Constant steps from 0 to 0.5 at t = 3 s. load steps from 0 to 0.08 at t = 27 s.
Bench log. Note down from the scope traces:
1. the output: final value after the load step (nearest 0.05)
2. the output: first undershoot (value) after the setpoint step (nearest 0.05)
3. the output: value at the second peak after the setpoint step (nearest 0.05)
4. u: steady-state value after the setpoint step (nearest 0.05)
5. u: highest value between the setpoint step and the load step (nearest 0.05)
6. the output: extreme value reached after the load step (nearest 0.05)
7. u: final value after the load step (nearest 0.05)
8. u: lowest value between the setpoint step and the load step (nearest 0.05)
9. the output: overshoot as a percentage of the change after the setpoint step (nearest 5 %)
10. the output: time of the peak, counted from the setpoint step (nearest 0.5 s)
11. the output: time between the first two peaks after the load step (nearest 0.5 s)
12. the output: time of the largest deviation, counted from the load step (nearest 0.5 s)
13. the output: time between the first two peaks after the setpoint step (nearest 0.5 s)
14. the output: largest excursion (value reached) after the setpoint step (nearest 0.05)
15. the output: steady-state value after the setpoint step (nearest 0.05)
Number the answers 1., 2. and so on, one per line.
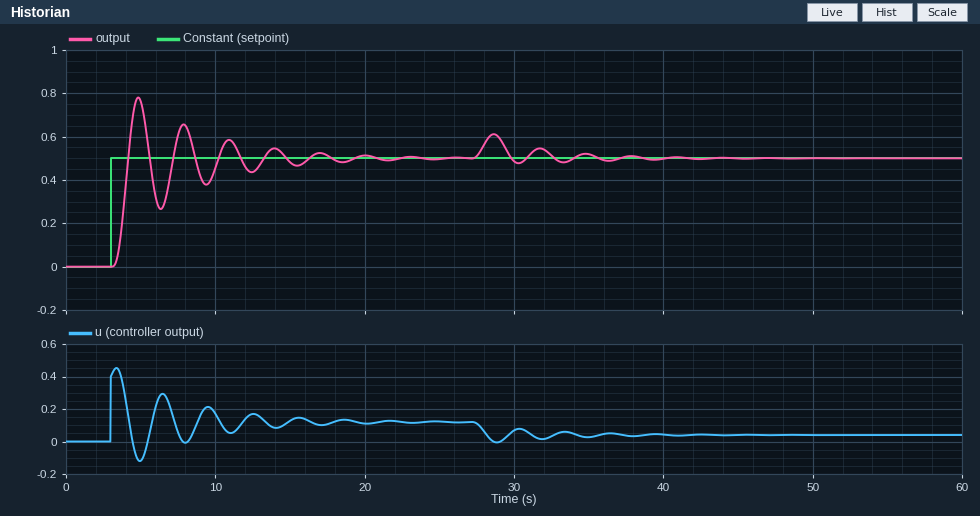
1. 0.50
2. 0.25
3. 0.65
4. 0.10
5. 0.45
6. 0.60
7. 0.05
8. -0.10
9. 55 %
10. 2.0 s
11. 3.0 s
12. 1.5 s
13. 3.0 s
14. 0.80
15. 0.50
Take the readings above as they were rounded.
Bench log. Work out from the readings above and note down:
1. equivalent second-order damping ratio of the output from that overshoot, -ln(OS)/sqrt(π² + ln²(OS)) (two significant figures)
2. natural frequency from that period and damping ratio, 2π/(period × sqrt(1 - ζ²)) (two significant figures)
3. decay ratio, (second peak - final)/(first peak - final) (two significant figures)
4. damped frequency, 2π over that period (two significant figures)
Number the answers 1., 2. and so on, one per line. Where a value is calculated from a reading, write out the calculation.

1. ln(0.55) = -0.598; 0.598 / sqrt(9.870 + 0.357) = 0.19
2. 2π / (3 × sqrt(1 - 0.19²)) = 2.1 rad/s
3. (0.65 - 0.5) / (0.8 - 0.5) = 0.50
4. 2π / 3 = 2.1 rad/s
